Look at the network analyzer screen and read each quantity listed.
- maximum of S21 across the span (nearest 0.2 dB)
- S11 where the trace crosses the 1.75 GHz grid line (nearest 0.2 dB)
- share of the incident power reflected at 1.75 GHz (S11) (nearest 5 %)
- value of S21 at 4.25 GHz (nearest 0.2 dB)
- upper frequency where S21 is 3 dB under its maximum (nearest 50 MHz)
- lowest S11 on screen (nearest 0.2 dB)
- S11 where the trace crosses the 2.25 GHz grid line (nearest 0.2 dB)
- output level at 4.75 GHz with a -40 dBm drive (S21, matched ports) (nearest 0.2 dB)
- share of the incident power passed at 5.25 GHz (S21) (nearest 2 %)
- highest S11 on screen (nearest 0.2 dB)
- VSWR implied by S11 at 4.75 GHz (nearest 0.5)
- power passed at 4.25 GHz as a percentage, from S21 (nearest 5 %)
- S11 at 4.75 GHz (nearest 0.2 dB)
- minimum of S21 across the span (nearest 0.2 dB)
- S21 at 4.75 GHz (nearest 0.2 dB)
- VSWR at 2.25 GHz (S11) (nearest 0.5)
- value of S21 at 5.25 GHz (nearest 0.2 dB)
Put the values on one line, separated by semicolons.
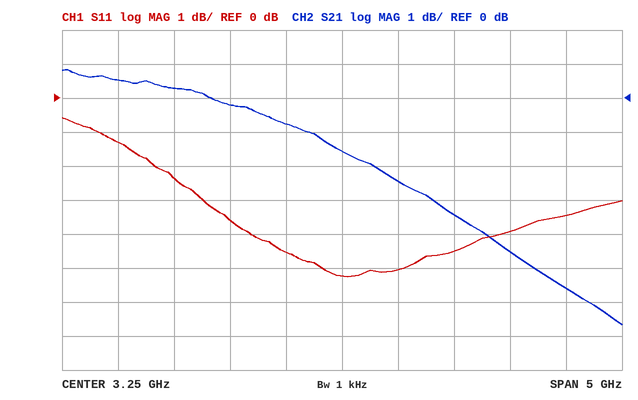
0.8 dB; -2.4 dB; 60 %; -3.4 dB; 3.60 GHz; -5.2 dB; -3.6 dB; -44.6 dBm; 28 %; -0.6 dB; 4.5; 45 %; -4.0 dB; -6.6 dB; -4.6 dB; 5.0; -5.6 dB
